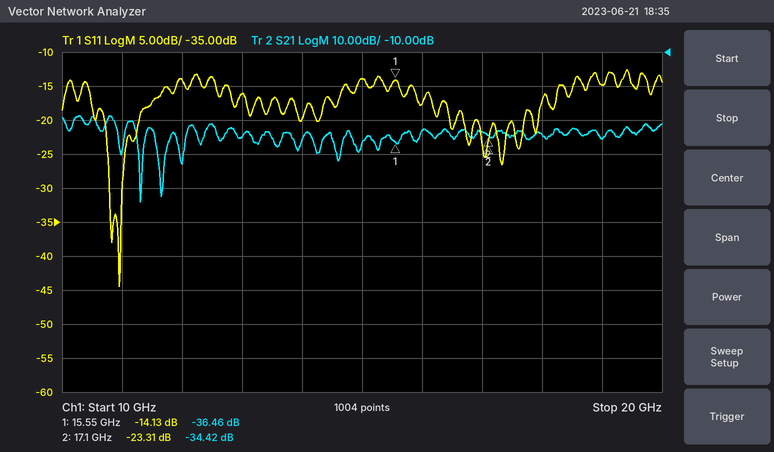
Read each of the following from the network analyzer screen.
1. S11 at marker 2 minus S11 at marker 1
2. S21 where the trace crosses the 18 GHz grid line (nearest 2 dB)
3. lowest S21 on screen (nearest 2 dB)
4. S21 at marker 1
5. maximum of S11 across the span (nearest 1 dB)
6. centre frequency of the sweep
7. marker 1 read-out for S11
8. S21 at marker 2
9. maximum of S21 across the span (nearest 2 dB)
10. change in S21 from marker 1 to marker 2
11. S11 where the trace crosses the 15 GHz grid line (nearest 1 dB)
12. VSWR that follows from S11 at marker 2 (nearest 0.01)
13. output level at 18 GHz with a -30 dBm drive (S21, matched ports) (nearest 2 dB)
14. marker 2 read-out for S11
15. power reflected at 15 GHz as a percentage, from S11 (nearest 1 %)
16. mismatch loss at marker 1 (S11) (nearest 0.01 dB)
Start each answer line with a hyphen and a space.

- -9.18 dB
- -34 dB
- -54 dB
- -36.46 dB
- -13 dB
- 15 GHz
- -14.13 dB
- -34.42 dB
- -28 dB
- 2.04 dB
- -14 dB
- 1.15
- -64 dBm
- -23.31 dB
- 4 %
- 0.17 dB
